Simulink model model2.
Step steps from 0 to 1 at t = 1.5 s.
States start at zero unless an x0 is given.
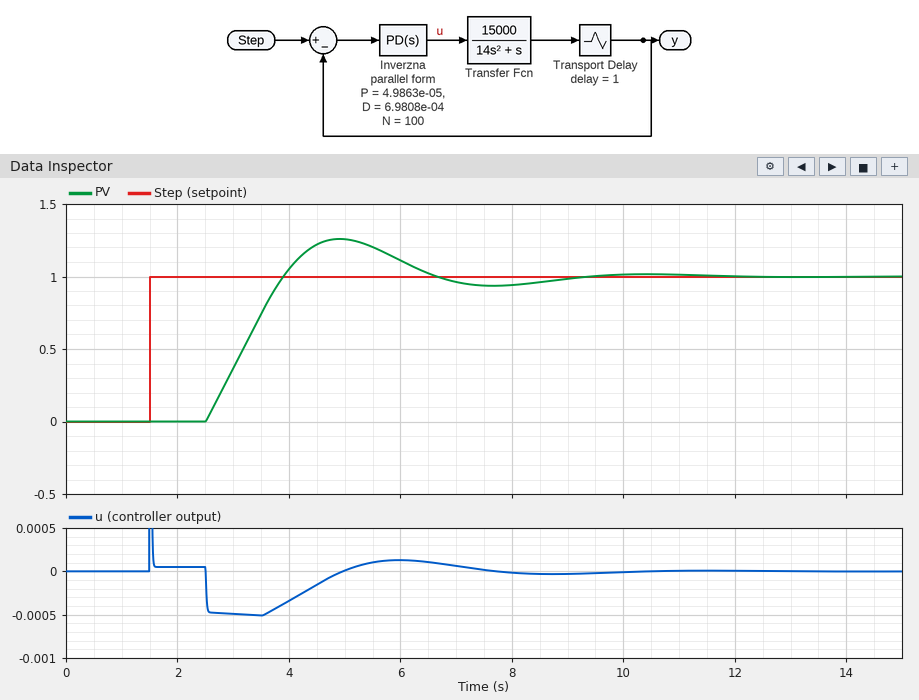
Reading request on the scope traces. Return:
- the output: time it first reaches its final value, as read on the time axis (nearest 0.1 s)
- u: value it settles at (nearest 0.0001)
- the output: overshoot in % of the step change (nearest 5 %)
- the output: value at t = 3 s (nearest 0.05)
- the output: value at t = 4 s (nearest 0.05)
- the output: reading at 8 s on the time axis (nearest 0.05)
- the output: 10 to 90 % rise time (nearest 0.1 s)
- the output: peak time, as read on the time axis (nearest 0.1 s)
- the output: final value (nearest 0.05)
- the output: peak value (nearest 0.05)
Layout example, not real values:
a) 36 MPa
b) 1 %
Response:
a) 3.9 s
b) 0.0000
c) 25 %
d) 0.35
e) 1.05
f) 0.95
g) 1.1 s
h) 4.9 s
i) 1.00
j) 1.25
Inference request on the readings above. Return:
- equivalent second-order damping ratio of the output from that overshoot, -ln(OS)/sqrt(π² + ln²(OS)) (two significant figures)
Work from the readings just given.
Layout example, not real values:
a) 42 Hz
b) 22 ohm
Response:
a) 0.40
